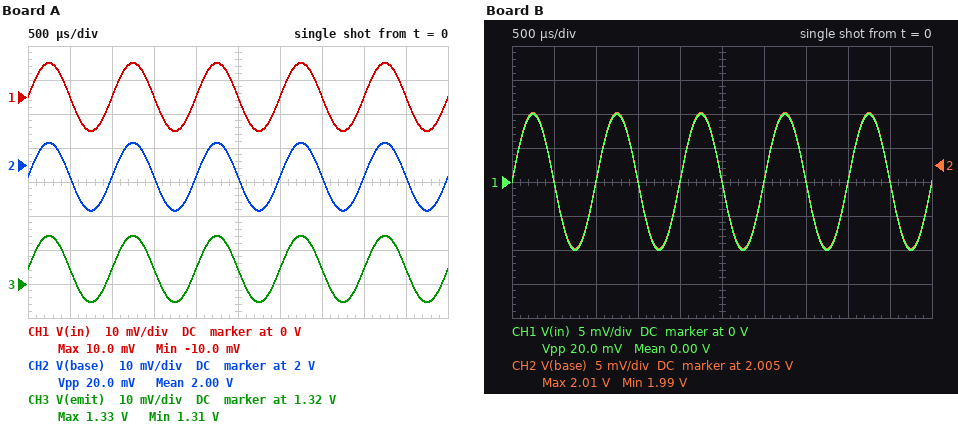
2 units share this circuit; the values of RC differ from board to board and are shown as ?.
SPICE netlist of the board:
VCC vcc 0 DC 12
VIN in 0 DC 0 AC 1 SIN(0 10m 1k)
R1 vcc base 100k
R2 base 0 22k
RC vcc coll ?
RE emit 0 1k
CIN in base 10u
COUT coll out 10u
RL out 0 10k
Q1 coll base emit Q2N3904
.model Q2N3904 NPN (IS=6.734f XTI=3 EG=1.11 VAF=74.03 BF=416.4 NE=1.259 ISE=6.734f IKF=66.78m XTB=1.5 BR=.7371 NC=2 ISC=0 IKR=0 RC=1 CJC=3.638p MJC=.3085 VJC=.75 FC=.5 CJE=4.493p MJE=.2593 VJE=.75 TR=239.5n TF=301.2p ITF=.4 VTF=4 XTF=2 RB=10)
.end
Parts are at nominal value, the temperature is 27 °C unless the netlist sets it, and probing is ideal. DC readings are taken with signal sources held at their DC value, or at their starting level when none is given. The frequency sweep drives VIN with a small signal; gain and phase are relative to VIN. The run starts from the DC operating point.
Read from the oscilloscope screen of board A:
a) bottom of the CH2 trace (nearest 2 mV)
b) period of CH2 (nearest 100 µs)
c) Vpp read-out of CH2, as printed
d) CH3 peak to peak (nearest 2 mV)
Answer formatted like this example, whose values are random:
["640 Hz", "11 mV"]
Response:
["1.986 V", "1.0 ms", "20.0 mV", "20 mV"]
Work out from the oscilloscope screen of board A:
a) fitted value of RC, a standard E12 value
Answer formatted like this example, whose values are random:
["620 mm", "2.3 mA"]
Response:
["5.6 kΩ"]
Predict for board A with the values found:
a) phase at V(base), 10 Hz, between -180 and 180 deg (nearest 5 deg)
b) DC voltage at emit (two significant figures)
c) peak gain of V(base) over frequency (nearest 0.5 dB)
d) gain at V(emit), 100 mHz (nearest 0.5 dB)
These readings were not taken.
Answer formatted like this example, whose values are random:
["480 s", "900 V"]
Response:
["5 deg", "1.3 V", "0 dB", "-20.0 dB"]
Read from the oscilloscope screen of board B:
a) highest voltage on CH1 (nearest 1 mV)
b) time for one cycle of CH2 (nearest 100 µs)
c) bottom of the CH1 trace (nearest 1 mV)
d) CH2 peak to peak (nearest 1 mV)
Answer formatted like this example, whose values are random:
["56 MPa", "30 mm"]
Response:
["10 mV", "1.0 ms", "-10 mV", "20 mV"]
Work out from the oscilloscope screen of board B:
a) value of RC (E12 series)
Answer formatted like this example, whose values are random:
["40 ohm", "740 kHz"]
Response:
["2.7 kΩ"]
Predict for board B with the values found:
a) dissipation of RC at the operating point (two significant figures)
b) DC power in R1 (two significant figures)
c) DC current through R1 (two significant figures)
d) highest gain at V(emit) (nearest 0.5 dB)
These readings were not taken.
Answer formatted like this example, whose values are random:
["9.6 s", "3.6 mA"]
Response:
["4.7 mW", "1.0 mW", "100 µA", "0 dB"]
